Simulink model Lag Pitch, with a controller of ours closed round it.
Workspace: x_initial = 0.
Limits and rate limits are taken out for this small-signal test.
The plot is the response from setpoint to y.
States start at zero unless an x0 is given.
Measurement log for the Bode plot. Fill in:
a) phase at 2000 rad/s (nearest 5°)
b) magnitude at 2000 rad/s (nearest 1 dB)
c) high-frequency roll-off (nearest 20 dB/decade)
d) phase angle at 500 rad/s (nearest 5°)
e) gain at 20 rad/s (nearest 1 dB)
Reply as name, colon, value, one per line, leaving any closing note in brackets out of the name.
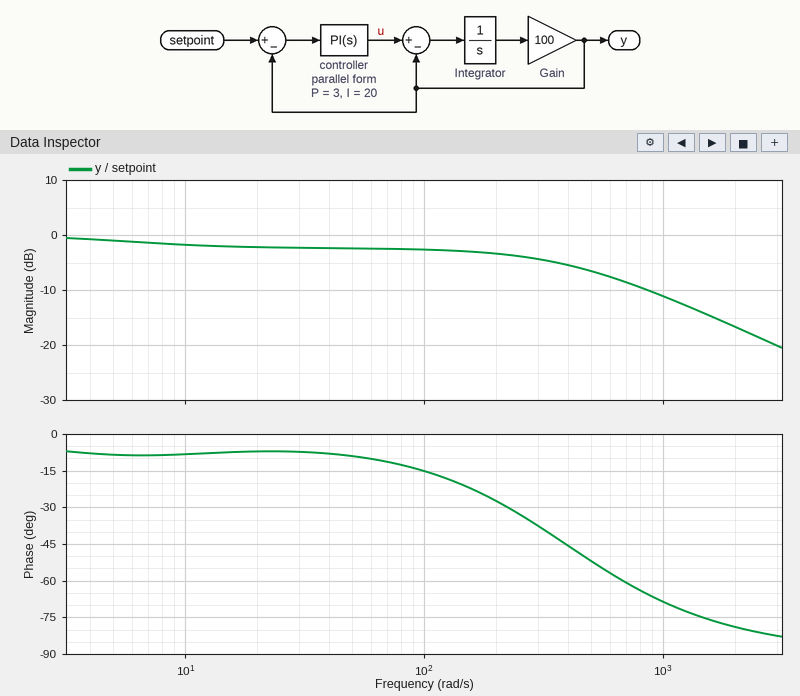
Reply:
phase at 2000 rad/s: -80°
magnitude at 2000 rad/s: -17 dB
high-frequency roll-off: -20 dB/decade
phase angle at 500 rad/s: -50°
gain at 20 rad/s: -2 dB
